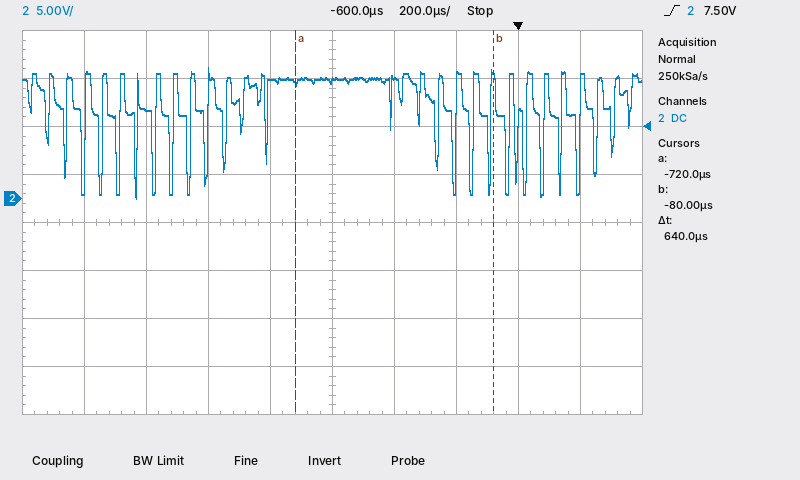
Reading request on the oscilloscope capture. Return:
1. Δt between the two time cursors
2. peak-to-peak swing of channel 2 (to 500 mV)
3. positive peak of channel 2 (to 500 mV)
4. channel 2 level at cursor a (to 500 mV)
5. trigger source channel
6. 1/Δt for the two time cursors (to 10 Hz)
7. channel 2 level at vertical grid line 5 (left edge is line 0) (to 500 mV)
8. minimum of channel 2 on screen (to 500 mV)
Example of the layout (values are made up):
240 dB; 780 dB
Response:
640 µs; 13.5 V; 13.5 V; 12.0 V; channel 2; 1.56 kHz; 12.5 V; 0.0 V
